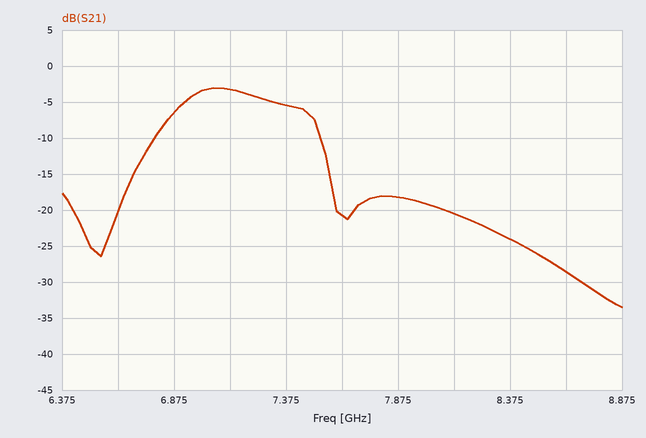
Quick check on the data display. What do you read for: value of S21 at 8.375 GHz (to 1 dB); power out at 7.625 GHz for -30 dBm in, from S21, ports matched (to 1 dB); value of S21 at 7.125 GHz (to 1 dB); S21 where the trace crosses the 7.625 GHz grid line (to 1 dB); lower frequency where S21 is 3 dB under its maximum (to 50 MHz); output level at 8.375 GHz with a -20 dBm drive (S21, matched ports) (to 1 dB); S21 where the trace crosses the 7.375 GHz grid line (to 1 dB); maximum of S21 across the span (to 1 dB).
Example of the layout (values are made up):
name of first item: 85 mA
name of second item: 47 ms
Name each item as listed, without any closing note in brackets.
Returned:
value of S21 at 8.375 GHz: -24 dB
power out at 7.625 GHz for -30 dBm in, from S21, ports matched: -51 dBm
value of S21 at 7.125 GHz: -3 dB
S21 where the trace crosses the 7.625 GHz grid line: -21 dB
lower frequency where S21 is 3 dB under its maximum: 6.90 GHz
output level at 8.375 GHz with a -20 dBm drive (S21, matched ports): -44 dBm
S21 where the trace crosses the 7.375 GHz grid line: -5 dB
maximum of S21 across the span: -3 dB
